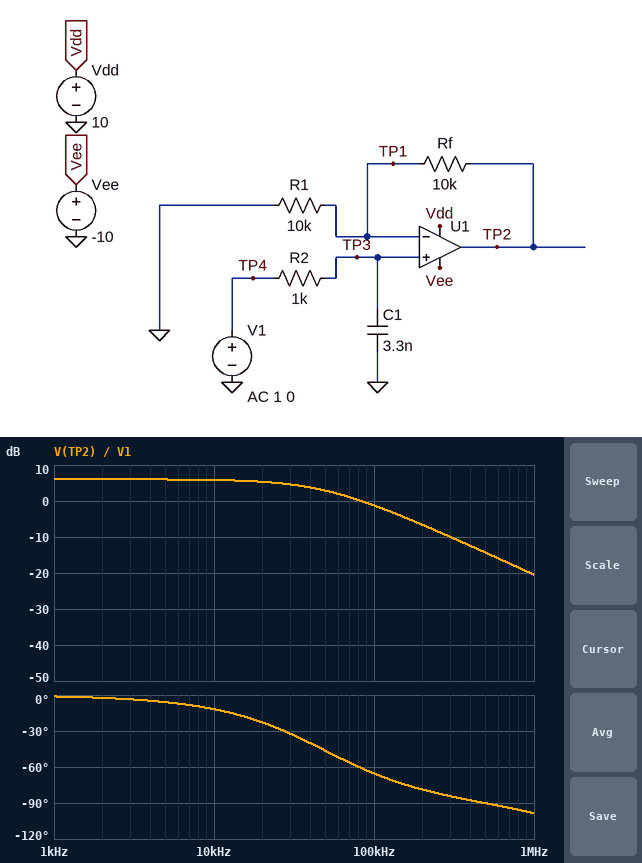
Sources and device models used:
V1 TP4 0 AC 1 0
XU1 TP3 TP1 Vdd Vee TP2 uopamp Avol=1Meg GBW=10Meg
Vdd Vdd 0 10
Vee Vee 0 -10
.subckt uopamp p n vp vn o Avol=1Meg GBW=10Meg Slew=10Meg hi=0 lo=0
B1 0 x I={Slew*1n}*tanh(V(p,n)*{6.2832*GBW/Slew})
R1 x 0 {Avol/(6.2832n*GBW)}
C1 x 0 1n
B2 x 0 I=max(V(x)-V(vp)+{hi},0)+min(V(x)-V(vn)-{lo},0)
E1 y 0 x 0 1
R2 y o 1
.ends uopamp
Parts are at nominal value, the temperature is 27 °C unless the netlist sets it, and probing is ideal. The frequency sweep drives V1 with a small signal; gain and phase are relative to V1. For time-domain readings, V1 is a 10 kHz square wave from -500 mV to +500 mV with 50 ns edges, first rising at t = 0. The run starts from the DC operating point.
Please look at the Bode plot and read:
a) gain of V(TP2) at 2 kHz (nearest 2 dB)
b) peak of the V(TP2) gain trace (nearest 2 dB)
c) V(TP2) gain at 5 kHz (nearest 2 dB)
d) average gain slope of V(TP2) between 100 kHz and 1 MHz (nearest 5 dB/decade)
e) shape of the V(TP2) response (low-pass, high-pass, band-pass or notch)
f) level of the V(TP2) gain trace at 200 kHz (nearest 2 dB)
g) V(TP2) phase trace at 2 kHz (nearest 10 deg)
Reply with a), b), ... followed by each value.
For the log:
a) 6 dB
b) 6 dB
c) 6 dB
d) -20 dB/decade
e) low-pass
f) -6 dB
g) 0 deg
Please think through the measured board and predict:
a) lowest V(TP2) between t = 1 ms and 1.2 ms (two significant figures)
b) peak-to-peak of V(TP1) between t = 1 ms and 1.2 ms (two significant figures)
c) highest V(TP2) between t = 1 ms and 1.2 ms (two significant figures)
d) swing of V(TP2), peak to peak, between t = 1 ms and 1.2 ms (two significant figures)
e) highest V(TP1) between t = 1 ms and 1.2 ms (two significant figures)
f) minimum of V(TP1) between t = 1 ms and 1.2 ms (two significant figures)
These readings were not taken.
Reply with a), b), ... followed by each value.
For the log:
a) -1.0 V
b) 1.0 V
c) 1.0 V
d) 2.0 V
e) 500 mV
f) -500 mV
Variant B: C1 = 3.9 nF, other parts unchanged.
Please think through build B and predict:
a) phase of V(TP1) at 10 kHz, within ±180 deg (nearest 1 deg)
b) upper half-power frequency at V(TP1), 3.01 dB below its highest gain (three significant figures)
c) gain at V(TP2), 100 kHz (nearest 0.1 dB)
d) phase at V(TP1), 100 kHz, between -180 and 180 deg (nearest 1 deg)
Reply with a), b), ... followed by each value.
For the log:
a) -14 deg
b) 40.8 kHz
c) -2.4 dB
d) -69 deg
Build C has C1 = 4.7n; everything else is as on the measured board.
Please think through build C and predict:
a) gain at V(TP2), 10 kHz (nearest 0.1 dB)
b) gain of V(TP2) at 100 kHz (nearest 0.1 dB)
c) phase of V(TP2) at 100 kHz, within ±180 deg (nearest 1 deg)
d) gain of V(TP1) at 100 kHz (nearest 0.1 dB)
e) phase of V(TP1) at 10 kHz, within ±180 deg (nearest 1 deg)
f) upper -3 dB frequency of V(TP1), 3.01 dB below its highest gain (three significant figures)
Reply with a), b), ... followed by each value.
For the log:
a) 5.7 dB
b) -3.9 dB
c) -72 deg
d) -9.9 dB
e) -17 deg
f) 33.9 kHz
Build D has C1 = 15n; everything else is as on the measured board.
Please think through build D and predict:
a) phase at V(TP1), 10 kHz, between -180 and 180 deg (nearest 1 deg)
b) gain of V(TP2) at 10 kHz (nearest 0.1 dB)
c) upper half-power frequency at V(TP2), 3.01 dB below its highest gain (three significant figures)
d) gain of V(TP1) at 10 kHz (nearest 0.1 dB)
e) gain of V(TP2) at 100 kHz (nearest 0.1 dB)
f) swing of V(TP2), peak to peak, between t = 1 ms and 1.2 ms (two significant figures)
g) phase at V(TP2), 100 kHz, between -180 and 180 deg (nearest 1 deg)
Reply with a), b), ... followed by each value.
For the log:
a) -43 deg
b) 3.3 dB
c) 10.6 kHz
d) -2.8 dB
e) -13.5 dB
f) 1.9 V
g) -85 deg
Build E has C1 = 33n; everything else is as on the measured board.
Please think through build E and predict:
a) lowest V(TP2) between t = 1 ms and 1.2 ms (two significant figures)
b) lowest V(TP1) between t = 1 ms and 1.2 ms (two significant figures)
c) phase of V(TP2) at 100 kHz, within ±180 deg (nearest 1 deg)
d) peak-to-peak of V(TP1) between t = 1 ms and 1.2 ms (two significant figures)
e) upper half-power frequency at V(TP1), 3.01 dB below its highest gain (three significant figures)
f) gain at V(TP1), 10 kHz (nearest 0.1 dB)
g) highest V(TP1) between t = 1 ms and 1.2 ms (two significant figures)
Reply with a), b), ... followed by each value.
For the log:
a) -640 mV
b) -320 mV
c) -88 deg
d) 640 mV
e) 4.82 kHz
f) -7.2 dB
g) 320 mV
